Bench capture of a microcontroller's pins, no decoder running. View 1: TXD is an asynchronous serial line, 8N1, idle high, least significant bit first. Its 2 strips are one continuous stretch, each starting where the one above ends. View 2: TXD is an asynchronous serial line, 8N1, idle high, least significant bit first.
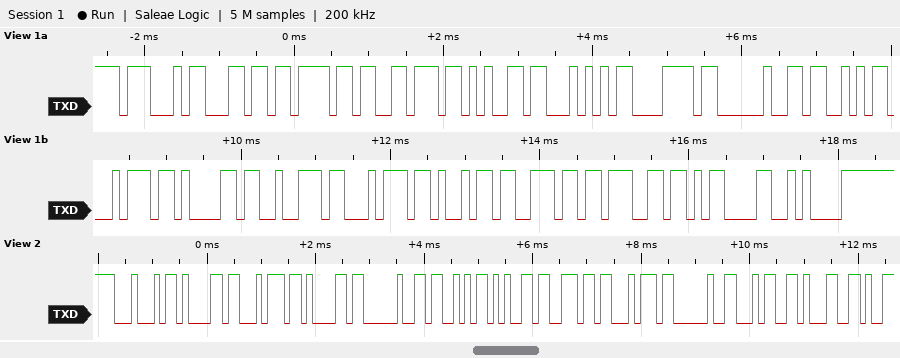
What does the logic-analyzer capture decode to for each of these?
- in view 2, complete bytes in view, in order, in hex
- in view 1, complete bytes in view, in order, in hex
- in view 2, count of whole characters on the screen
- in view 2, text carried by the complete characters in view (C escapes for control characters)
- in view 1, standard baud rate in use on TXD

44 61 74 61 20 53 65 6E 74 20 34 31
47 6C 6F 76 65 54 78 20 53 74 61 72 74 69 6E 67 0D 0A
12
"Data Sent 41"
9600 baud
